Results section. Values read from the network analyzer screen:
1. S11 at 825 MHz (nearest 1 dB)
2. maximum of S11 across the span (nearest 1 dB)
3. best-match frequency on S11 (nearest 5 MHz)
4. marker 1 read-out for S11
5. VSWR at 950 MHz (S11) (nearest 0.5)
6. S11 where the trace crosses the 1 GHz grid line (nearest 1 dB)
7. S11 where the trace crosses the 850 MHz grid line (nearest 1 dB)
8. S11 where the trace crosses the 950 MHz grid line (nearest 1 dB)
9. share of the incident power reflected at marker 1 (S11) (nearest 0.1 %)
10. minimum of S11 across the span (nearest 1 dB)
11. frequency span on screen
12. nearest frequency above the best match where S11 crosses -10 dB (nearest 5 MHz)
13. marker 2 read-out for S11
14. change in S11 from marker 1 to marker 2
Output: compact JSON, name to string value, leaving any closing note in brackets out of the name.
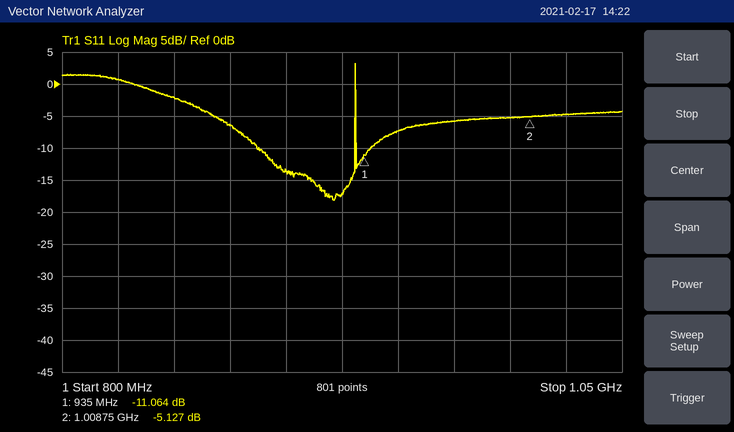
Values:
{"S11 at 825 MHz": "1 dB", "maximum of S11 across the span": "3 dB", "best-match frequency on S11": "920 MHz", "marker 1 read-out for S11": "-11.064 dB", "VSWR at 950 MHz (S11)": "2.5", "S11 where the trace crosses the 1 GHz grid line": "-5 dB", "S11 where the trace crosses the 850 MHz grid line": "-2 dB", "S11 where the trace crosses the 950 MHz grid line": "-7 dB", "share of the incident power reflected at marker 1 (S11)": "7.8 %", "minimum of S11 across the span": "-18 dB", "frequency span on screen": "250 MHz", "nearest frequency above the best match where S11 crosses -10 dB": "930 MHz", "marker 2 read-out for S11": "-5.127 dB", "change in S11 from marker 1 to marker 2": "5.937 dB"}
